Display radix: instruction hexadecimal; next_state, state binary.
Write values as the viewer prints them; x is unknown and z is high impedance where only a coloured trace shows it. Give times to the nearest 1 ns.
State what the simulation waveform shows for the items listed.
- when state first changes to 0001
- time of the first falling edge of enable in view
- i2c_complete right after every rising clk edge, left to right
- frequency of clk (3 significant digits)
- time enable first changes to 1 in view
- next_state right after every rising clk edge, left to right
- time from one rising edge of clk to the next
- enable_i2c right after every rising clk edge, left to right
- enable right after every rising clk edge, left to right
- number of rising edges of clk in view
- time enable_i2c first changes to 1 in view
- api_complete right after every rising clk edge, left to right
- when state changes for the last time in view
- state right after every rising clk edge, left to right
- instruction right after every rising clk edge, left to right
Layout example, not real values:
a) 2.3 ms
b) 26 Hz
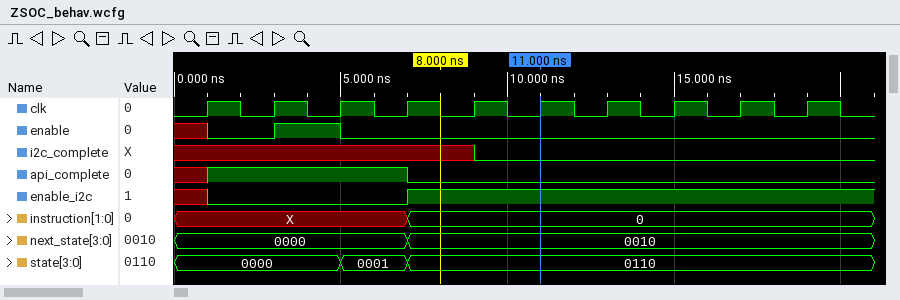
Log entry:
a) 5 ns
b) 5 ns
c) x x x x 0 0 0 0 0 0
d) 500 MHz
e) 3 ns
f) 0000, 0000, 0000, 0010, 0010, 0010, 0010, 0010, 0010, 0010
g) 2 ns
h) 0 0 0 1 1 1 1 1 1 1
i) 0 1 0 0 0 0 0 0 0 0
j) 10
k) 7 ns
l) 1 1 1 0 0 0 0 0 0 0
m) 7 ns
n) 0000, 0000, 0001, 0110, 0110, 0110, 0110, 0110, 0110, 0110
o) X, X, X, 0, 0, 0, 0, 0, 0, 0
